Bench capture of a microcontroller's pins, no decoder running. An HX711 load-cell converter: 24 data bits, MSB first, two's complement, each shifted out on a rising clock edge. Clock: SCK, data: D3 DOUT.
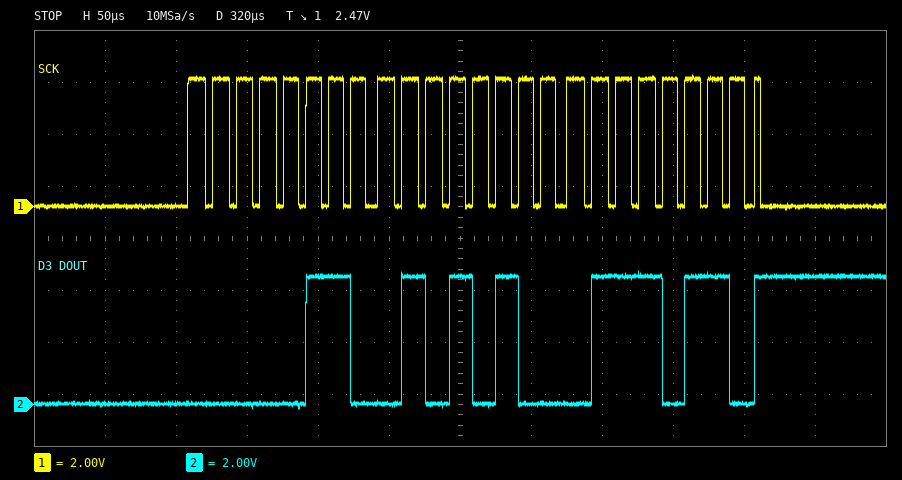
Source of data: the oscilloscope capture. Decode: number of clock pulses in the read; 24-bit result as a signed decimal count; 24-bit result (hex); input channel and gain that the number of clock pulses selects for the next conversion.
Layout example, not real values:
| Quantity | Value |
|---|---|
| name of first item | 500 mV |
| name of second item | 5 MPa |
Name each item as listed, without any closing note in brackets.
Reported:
| Quantity | Value |
|---|---|
| number of clock pulses in the read | 25 |
| 24-bit result as a signed decimal count | 414838 |
| 24-bit result | 0x065476 |
| input channel and gain that the number of clock pulses selects for the next conversion | channel A, gain 128 |
